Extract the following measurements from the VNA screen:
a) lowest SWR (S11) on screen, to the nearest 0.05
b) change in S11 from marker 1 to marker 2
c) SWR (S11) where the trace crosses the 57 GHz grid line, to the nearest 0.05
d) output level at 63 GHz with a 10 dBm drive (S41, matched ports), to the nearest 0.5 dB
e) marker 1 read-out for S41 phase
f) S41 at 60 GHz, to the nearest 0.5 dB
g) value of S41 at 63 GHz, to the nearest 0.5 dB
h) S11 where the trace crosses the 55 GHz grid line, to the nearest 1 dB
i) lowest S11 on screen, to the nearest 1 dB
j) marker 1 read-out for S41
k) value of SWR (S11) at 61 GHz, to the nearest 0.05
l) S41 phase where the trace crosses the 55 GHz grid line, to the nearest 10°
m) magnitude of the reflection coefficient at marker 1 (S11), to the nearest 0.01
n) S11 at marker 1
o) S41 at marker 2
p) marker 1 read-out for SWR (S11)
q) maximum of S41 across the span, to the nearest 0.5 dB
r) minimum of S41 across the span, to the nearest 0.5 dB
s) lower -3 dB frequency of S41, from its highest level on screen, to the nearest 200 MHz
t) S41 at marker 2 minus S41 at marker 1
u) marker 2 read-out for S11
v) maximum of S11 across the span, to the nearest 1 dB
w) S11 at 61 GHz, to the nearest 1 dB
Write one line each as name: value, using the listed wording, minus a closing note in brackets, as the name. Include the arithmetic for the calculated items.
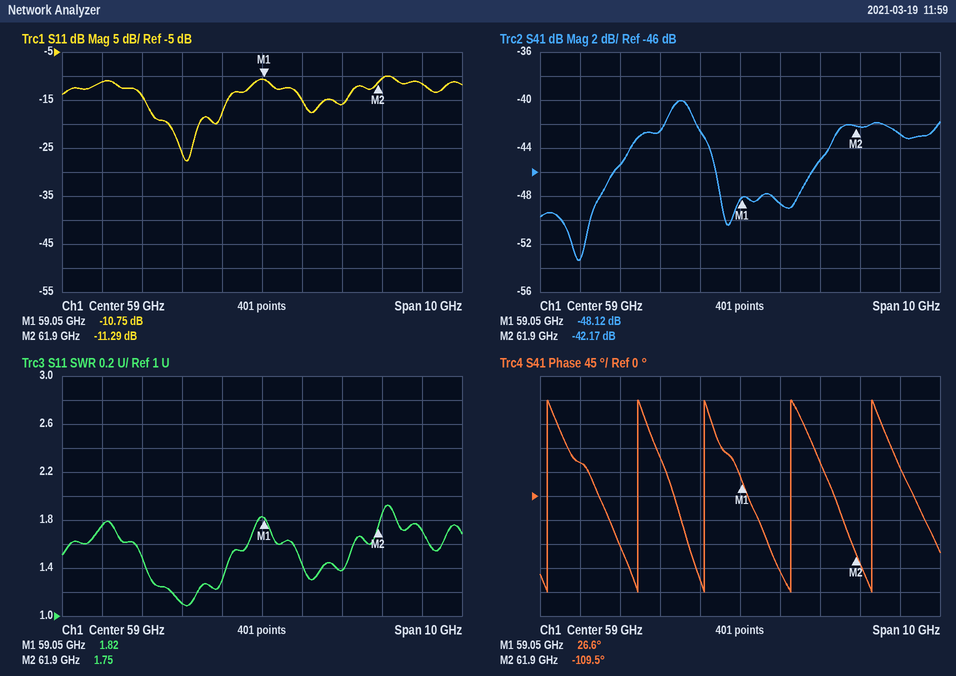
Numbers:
lowest SWR (S11) on screen, to the nearest 0.05: 1.10
change in S11 from marker 1 to marker 2: -11.29 − (-10.75) = -0.54 dB
SWR (S11) where the trace crosses the 57 GHz grid line, to the nearest 0.05: 1.10
output level at 63 GHz with a 10 dBm drive (S41, matched ports), to the nearest 0.5 dB: 10 dBm + (-43.0 dB) = -33.0 dBm
marker 1 read-out for S41 phase: 26.6°
S41 at 60 GHz, to the nearest 0.5 dB: -48.5 dB
value of S41 at 63 GHz, to the nearest 0.5 dB: -43.0 dB
S11 where the trace crosses the 55 GHz grid line, to the nearest 1 dB: -11 dB
lowest S11 on screen, to the nearest 1 dB: -28 dB
marker 1 read-out for S41: -48.12 dB
value of SWR (S11) at 61 GHz, to the nearest 0.05: 1.40
S41 phase where the trace crosses the 55 GHz grid line, to the nearest 10°: 60°
magnitude of the reflection coefficient at marker 1 (S11), to the nearest 0.01: 10^(-10.75/20) ≈ 0.29
S11 at marker 1: -10.75 dB
S41 at marker 2: -42.17 dB
marker 1 read-out for SWR: 1.82
maximum of S41 across the span, to the nearest 0.5 dB: -40.0 dB
minimum of S41 across the span, to the nearest 0.5 dB: -53.5 dB
lower -3 dB frequency of S41, from its highest level on screen, to the nearest 200 MHz: 56.4 GHz
S41 at marker 2 minus S41 at marker 1: -42.17 − (-48.12) = 5.95 dB
marker 2 read-out for S11: -11.29 dB
maximum of S11 across the span, to the nearest 1 dB: -10 dB
S11 at 61 GHz, to the nearest 1 dB: -16 dB
